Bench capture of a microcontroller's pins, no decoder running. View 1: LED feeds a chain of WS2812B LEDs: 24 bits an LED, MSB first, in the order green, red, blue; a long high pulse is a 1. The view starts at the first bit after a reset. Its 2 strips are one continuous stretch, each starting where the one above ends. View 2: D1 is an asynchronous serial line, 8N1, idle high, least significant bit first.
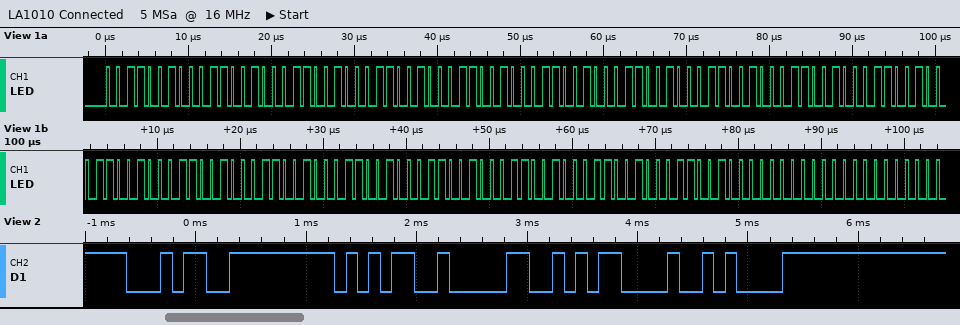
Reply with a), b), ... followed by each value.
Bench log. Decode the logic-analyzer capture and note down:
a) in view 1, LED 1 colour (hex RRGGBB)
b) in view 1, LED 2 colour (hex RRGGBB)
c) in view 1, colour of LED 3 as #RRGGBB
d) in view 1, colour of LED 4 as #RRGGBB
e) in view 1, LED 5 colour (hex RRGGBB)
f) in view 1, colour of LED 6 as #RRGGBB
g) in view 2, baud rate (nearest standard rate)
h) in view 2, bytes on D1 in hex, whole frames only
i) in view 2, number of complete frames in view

a) #323232
b) #323232
c) #323232
d) #323232
e) #323232
f) #323232
g) 9600 baud
h) 34 35 30 0D 0A
i) 5
